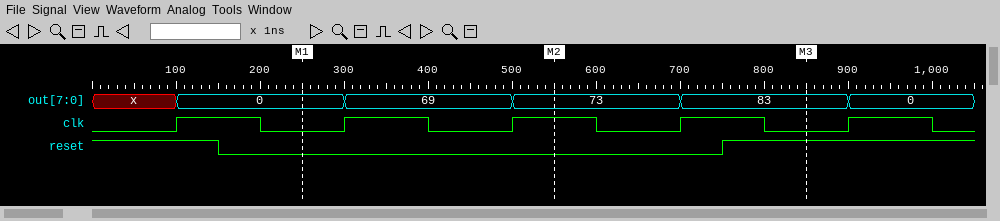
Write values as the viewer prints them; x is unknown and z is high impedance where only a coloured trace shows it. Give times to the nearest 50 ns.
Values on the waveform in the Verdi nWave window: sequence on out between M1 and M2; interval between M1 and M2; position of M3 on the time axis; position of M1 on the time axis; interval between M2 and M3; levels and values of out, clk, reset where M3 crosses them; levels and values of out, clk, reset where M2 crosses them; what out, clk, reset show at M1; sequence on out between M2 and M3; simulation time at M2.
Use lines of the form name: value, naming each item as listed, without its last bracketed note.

sequence on out between M1 and M2: 0, 69, 73
interval between M1 and M2: 300 ns
position of M3 on the time axis: 850 ns
position of M1 on the time axis: 250 ns
interval between M2 and M3: 300 ns
levels and values of out, clk, reset where M3 crosses them: out=83, clk=0, reset=1
levels and values of out, clk, reset where M2 crosses them: out=73, clk=1, reset=0
what out, clk, reset show at M1: out=0, clk=0, reset=0
sequence on out between M2 and M3: 73, 83
simulation time at M2: 550 ns
